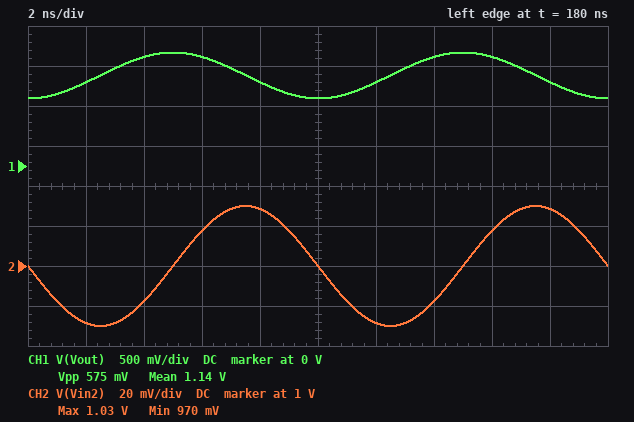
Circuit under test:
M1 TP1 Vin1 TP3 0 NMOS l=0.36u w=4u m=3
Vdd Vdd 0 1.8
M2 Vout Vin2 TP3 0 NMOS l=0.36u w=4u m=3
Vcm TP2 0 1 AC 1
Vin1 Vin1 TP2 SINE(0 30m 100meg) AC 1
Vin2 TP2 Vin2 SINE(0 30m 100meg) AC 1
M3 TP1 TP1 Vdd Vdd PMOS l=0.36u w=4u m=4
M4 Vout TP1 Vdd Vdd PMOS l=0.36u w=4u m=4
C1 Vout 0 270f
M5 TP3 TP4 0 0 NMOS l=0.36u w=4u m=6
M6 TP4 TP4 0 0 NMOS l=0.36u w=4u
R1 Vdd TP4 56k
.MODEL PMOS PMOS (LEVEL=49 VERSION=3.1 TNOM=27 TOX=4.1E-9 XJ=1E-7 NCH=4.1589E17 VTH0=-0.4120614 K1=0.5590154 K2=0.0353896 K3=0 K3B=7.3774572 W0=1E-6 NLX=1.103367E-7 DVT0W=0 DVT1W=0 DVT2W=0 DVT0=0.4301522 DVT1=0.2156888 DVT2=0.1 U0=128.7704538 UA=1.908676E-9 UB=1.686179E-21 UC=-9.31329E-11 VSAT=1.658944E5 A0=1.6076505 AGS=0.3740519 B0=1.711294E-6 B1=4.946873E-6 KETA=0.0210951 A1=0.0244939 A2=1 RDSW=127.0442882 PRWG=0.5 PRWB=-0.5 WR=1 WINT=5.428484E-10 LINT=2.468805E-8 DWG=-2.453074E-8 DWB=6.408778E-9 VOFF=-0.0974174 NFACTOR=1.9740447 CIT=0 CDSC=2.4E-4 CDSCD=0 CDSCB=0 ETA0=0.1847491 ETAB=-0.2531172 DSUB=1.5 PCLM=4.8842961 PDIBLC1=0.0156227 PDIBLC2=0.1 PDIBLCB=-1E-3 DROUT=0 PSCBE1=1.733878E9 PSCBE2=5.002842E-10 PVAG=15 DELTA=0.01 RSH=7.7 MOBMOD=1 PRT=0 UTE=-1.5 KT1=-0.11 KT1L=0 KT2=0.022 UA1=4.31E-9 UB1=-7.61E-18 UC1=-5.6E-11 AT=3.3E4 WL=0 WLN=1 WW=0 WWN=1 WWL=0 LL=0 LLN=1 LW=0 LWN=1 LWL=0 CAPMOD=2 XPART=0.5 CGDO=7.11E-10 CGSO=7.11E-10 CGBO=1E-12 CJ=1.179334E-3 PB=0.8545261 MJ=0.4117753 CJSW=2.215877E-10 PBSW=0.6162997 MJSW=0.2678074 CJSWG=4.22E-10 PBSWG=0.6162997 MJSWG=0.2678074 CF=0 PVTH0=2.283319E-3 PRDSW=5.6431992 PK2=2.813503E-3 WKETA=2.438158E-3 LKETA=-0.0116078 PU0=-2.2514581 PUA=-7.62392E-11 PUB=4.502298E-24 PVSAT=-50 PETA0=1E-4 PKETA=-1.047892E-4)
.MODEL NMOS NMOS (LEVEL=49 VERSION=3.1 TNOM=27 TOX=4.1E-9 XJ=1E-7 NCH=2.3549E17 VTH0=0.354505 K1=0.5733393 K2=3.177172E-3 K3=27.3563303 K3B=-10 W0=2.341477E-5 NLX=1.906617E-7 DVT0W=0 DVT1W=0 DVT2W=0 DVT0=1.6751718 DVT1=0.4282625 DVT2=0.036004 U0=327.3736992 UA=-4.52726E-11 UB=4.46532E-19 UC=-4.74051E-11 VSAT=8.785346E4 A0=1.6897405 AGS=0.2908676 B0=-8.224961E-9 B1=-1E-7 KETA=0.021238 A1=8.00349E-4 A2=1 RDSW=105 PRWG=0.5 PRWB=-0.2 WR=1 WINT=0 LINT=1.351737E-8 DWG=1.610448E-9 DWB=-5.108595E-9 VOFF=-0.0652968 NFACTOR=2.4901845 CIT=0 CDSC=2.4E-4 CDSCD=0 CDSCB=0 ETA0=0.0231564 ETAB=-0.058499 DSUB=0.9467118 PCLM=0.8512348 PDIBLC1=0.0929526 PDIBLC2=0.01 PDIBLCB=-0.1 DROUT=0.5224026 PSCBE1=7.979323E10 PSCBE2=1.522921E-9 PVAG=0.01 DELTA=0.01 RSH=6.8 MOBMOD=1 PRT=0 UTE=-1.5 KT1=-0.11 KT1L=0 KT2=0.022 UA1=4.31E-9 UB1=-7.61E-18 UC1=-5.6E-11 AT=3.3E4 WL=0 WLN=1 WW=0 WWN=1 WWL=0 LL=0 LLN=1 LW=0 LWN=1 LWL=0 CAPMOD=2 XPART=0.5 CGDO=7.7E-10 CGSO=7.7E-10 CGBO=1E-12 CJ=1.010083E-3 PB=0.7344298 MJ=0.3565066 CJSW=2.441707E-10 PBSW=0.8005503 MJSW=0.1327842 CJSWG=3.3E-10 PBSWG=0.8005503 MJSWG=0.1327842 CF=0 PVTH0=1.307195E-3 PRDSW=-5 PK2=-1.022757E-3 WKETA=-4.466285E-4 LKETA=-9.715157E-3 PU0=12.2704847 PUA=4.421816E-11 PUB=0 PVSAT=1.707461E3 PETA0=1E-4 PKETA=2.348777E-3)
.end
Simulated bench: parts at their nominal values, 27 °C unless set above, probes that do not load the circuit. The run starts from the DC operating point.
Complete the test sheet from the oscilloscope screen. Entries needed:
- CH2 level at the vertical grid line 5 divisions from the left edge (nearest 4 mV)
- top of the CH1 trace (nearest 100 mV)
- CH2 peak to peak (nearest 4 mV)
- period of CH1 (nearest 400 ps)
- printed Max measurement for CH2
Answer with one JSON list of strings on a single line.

["1.000 V", "1.4 V", "60 mV", "10.0 ns", "1.03 V"]
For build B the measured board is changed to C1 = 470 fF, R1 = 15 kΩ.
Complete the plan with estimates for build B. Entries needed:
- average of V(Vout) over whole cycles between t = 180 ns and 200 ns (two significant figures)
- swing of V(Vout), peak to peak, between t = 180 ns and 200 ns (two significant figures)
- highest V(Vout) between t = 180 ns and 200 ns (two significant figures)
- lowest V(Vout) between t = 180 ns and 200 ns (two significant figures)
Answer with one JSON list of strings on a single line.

["960 mV", "670 mV", "1.3 V", "630 mV"]
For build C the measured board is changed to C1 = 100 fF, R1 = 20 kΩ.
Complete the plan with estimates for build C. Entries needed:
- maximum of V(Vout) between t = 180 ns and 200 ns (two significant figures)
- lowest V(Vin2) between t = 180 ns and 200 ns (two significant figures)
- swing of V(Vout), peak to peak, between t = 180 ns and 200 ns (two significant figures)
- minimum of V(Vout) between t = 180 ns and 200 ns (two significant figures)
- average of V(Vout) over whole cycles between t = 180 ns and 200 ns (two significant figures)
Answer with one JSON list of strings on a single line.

["1.7 V", "970 mV", "1.3 V", "330 mV", "1.0 V"]
